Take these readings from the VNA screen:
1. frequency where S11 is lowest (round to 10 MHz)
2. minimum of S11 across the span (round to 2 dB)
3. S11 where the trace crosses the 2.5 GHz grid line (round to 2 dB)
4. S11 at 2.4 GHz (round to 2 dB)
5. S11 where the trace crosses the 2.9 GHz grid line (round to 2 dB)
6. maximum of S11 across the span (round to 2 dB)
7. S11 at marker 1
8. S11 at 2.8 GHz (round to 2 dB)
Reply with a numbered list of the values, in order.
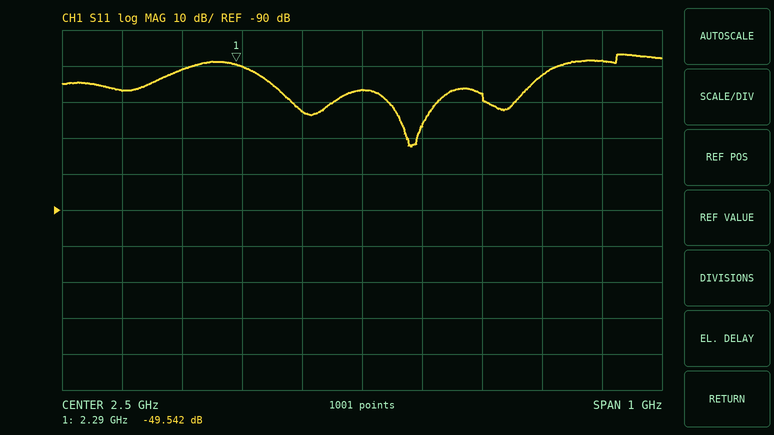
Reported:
1. 2.58 GHz
2. -72 dB
3. -56 dB
4. -62 dB
5. -48 dB
6. -46 dB
7. -49.542 dB
8. -52 dB
